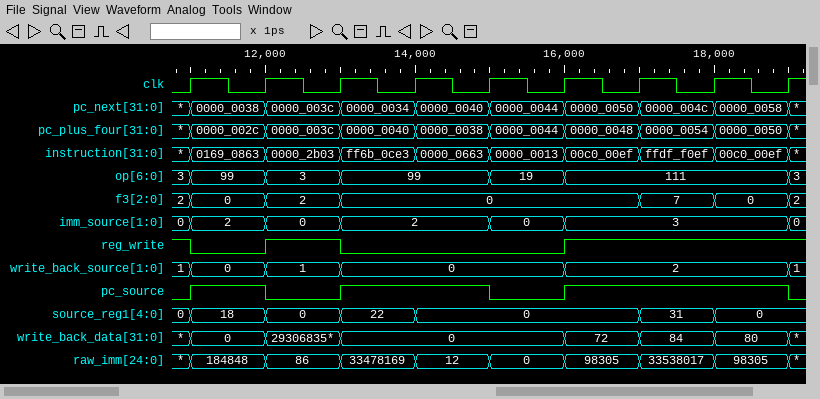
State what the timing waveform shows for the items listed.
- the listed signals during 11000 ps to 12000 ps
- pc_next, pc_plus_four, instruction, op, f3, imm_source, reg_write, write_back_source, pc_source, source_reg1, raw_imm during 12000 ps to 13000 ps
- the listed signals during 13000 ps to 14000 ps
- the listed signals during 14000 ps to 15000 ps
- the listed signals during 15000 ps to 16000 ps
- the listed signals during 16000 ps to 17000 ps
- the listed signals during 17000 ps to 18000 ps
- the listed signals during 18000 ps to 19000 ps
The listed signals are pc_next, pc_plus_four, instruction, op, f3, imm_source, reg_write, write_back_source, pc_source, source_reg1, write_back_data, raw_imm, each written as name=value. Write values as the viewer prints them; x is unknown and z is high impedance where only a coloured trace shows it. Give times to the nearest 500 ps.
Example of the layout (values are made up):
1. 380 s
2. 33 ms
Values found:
1. pc_next=0000_0038, pc_plus_four=0000_002c, instruction=0169_0863, op=99, f3=0, imm_source=2, reg_write=0, write_back_source=0, pc_source=1, source_reg1=18, write_back_data=0, raw_imm=184848
2. pc_next=0000_003c, pc_plus_four=0000_003c, instruction=0000_2b03, op=3, f3=2, imm_source=0, reg_write=1, write_back_source=1, pc_source=0, source_reg1=0, raw_imm=86
3. pc_next=0000_0034, pc_plus_four=0000_0040, instruction=ff6b_0ce3, op=99, f3=0, imm_source=2, reg_write=0, write_back_source=0, pc_source=1, source_reg1=22, write_back_data=0, raw_imm=33478169
4. pc_next=0000_0040, pc_plus_four=0000_0038, instruction=0000_0663, op=99, f3=0, imm_source=2, reg_write=0, write_back_source=0, pc_source=1, source_reg1=0, write_back_data=0, raw_imm=12
5. pc_next=0000_0044, pc_plus_four=0000_0044, instruction=0000_0013, op=19, f3=0, imm_source=0, reg_write=0, write_back_source=0, pc_source=0, source_reg1=0, write_back_data=0, raw_imm=0
6. pc_next=0000_0050, pc_plus_four=0000_0048, instruction=00c0_00ef, op=111, f3=0, imm_source=3, reg_write=1, write_back_source=2, pc_source=1, source_reg1=0, write_back_data=72, raw_imm=98305
7. pc_next=0000_004c, pc_plus_four=0000_0054, instruction=ffdf_f0ef, op=111, f3=7, imm_source=3, reg_write=1, write_back_source=2, pc_source=1, source_reg1=31, write_back_data=84, raw_imm=33538017
8. pc_next=0000_0058, pc_plus_four=0000_0050, instruction=00c0_00ef, op=111, f3=0, imm_source=3, reg_write=1, write_back_source=2, pc_source=1, source_reg1=0, write_back_data=80, raw_imm=98305
